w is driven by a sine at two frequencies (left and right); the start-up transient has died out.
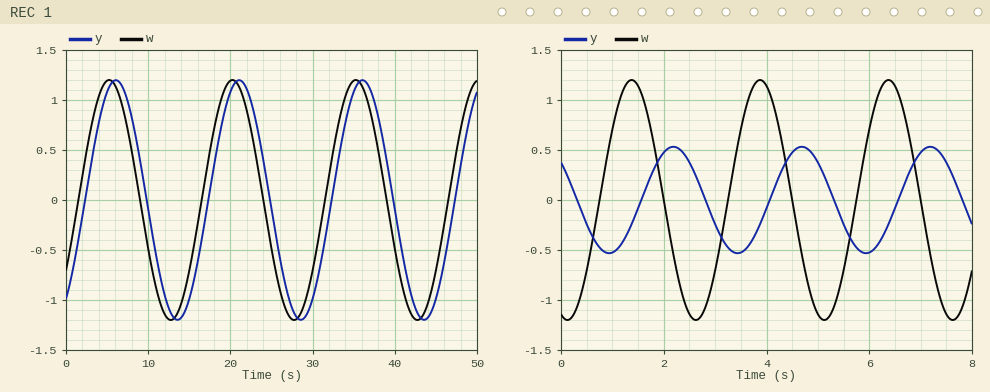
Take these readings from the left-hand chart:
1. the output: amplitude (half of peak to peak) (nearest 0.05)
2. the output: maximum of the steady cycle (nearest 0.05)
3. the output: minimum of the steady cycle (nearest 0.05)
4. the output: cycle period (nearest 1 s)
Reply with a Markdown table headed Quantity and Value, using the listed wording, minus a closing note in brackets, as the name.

| Quantity | Value |
|---|---|
| the output: amplitude (half of peak to peak) | 1.20 |
| the output: maximum of the steady cycle | 1.20 |
| the output: minimum of the steady cycle | -1.20 |
| the output: cycle period | 15 s |
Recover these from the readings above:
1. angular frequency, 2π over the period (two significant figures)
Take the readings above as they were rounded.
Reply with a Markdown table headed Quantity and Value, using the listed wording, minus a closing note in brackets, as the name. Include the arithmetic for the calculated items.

| Quantity | Value |
|---|---|
| angular frequency, 2π over the period | 2π / 15 = 0.42 rad/s |
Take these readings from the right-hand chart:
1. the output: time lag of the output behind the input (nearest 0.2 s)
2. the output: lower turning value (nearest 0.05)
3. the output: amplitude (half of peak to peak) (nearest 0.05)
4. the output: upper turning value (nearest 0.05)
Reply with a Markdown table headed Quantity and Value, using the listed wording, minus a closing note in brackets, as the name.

| Quantity | Value |
|---|---|
| the output: time lag of the output behind the input | 0.8 s |
| the output: lower turning value | -0.55 |
| the output: amplitude (half of peak to peak) | 0.55 |
| the output: upper turning value | 0.55 |
